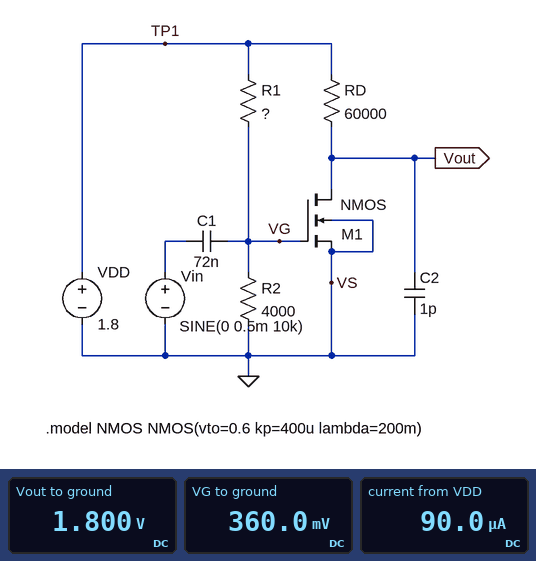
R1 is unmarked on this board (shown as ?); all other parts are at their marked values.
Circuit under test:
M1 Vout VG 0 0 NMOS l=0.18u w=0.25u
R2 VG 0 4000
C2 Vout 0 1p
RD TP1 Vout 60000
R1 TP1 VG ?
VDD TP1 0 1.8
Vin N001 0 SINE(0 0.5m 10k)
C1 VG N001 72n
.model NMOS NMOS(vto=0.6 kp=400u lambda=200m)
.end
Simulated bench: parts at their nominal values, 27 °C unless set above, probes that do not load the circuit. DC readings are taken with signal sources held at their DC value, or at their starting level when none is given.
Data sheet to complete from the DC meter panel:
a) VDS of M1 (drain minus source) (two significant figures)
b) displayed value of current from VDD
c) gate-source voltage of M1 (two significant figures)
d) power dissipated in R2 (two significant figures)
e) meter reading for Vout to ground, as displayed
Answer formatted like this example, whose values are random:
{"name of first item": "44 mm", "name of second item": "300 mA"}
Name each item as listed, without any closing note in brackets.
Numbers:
{"VDS of M1 (drain minus source)": "1.8 V", "displayed value of current from VDD": "90.0 µA", "gate-source voltage of M1": "360 mV", "power dissipated in R2": "32 µW", "meter reading for Vout to ground, as displayed": "1.800 V"}
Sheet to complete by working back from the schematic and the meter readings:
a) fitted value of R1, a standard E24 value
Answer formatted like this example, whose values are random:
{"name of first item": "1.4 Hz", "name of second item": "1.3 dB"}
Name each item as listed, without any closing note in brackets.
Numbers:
{"fitted value of R1, a standard E24 value": "16 kΩ"}
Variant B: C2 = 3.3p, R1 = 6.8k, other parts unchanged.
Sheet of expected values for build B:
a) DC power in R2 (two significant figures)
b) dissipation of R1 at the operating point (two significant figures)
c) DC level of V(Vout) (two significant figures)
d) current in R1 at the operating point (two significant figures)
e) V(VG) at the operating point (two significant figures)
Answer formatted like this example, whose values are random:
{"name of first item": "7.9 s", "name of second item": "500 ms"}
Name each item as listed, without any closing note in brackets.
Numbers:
{"DC power in R2": "110 µW", "dissipation of R1 at the operating point": "190 µW", "DC level of V(Vout)": "1.7 V", "current in R1 at the operating point": "170 µA", "V(VG) at the operating point": "670 mV"}
